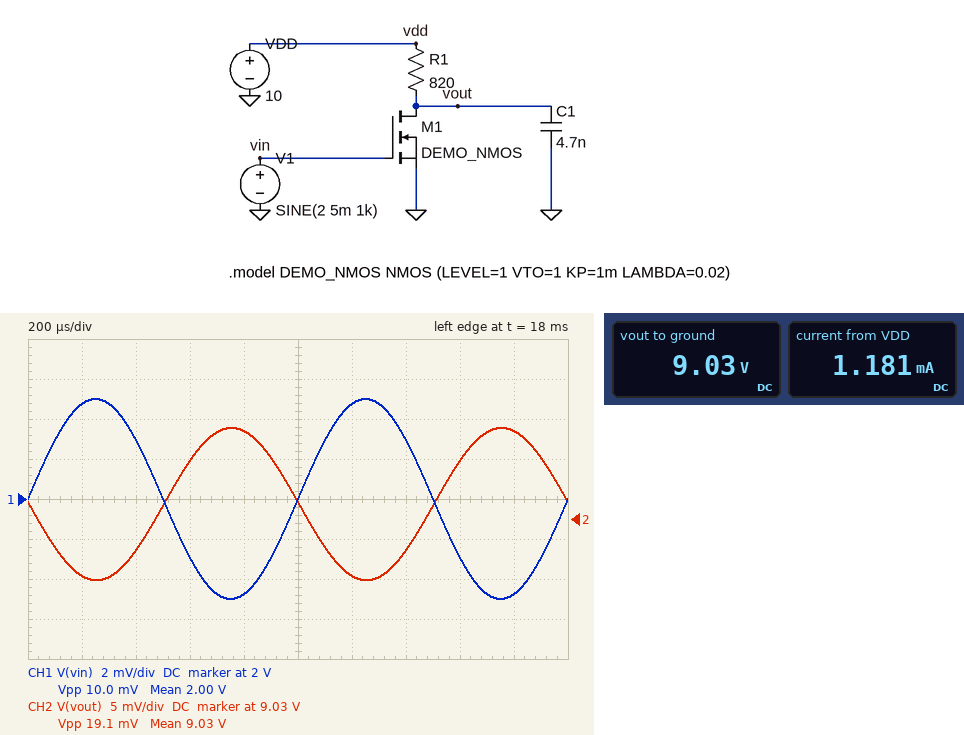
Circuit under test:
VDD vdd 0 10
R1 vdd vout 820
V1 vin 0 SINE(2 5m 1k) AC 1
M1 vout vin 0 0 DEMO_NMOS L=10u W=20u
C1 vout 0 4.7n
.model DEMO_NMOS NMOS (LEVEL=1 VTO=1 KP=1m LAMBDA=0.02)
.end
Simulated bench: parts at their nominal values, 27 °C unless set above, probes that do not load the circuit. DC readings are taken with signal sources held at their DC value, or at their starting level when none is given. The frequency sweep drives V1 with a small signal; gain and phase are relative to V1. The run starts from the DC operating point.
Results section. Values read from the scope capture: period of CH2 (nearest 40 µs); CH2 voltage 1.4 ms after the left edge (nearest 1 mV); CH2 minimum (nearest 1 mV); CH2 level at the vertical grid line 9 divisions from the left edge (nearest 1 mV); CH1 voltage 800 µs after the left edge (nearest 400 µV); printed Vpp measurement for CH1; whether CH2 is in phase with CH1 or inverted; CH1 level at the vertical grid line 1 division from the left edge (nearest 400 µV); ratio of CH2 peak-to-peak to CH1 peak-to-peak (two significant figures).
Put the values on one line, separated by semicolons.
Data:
1.00 ms; 9.026 V; 9.022 V; 9.041 V; 1.9952 V; 10.0 mV; inverted; 2.0048 V; 1.9
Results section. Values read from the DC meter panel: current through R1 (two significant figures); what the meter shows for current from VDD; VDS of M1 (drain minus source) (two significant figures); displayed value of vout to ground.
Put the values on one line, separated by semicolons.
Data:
1.2 mA; 1.181 mA; 9.0 V; 9.03 V
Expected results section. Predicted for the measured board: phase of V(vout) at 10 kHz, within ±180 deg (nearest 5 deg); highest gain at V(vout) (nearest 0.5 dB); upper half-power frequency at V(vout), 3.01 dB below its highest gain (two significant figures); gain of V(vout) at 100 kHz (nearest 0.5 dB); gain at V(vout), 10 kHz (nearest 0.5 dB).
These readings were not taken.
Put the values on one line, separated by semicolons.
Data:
165 deg; 5.5 dB; 42 kHz; -2.5 dB; 5.5 dB
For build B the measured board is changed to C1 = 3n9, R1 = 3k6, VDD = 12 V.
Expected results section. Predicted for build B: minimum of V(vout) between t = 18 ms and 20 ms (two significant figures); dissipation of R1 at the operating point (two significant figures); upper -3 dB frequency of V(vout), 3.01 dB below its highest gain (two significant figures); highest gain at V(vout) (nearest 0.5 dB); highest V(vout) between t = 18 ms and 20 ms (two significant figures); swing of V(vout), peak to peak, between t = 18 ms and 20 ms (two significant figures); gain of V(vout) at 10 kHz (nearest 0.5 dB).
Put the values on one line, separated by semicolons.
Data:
7.8 V; 4.8 mW; 12 kHz; 18.0 dB; 7.9 V; 77 mV; 15.5 dB
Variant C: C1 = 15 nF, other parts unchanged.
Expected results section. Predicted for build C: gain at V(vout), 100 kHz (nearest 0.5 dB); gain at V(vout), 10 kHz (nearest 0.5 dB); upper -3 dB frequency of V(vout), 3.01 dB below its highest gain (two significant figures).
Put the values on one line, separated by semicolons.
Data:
-12.0 dB; 3.5 dB; 13 kHz
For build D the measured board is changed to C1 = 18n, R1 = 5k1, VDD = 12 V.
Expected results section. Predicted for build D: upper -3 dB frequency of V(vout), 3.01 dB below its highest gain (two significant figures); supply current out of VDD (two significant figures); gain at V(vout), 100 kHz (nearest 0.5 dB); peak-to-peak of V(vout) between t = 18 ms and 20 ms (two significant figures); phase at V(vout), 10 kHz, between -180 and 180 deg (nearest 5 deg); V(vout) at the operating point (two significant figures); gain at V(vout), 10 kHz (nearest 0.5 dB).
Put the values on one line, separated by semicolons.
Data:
1.9 kHz; 1.1 mA; -14.0 dB; 92 mV; 100 deg; 6.3 V; 6.0 dB
